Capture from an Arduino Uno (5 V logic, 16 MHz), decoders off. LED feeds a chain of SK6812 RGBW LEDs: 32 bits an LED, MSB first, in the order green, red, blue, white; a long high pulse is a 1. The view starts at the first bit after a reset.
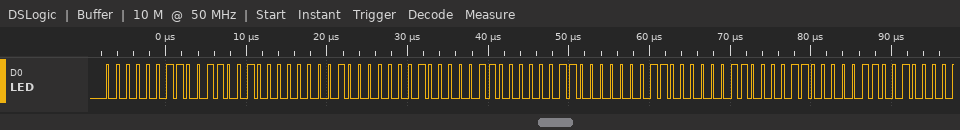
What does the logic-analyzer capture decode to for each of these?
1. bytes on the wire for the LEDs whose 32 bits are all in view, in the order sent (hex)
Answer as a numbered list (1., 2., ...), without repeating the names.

1. 03 32 01 01 06 06 03 03
